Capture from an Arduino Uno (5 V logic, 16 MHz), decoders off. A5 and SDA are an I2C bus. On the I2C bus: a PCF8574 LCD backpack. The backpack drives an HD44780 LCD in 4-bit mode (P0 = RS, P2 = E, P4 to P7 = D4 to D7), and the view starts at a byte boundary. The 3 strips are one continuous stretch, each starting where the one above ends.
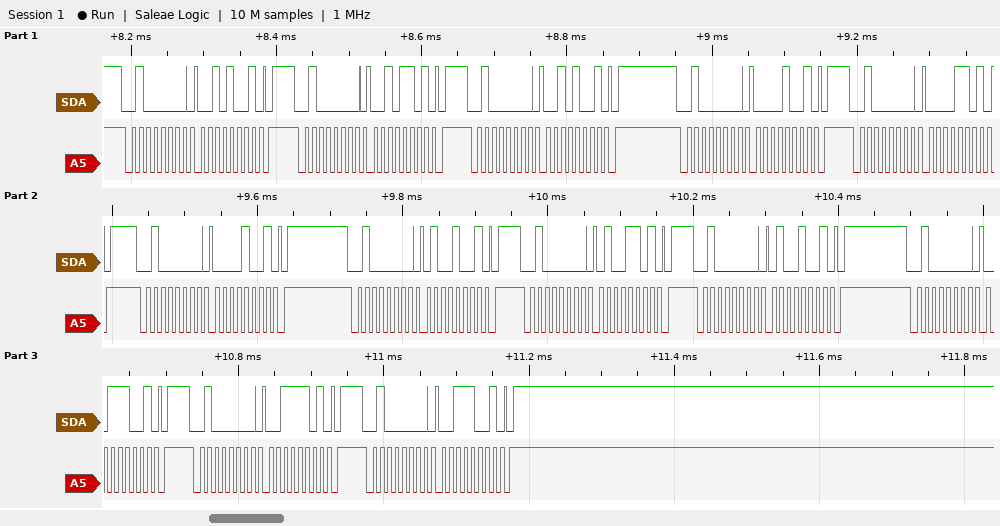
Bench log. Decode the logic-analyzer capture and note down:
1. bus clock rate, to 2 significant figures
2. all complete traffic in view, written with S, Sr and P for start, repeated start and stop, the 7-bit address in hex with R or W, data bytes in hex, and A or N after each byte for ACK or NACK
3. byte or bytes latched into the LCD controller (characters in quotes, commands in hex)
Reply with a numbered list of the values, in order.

1. 100 kHz
2. S 20W A 29 A P S 20W A 2D A P S 20W A 29 A P S 20W A 09 A P S 20W A 0D A P S 20W A 09 A P S 20W A 49 A P S 20W A 4D A P S 20W A 49 A P S 20W A 39 A P S 20W A 3D A P S 20W A 39 A P
3. ' ' 'C'
